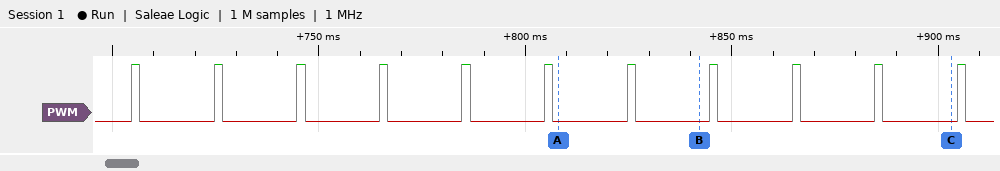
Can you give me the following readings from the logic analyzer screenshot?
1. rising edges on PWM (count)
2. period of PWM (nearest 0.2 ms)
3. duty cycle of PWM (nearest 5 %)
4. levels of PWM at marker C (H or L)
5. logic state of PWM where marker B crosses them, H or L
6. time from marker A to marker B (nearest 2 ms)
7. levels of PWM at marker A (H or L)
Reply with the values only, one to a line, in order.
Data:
11
20 ms
10 %
PWM=L
PWM=L
34 ms
PWM=L
